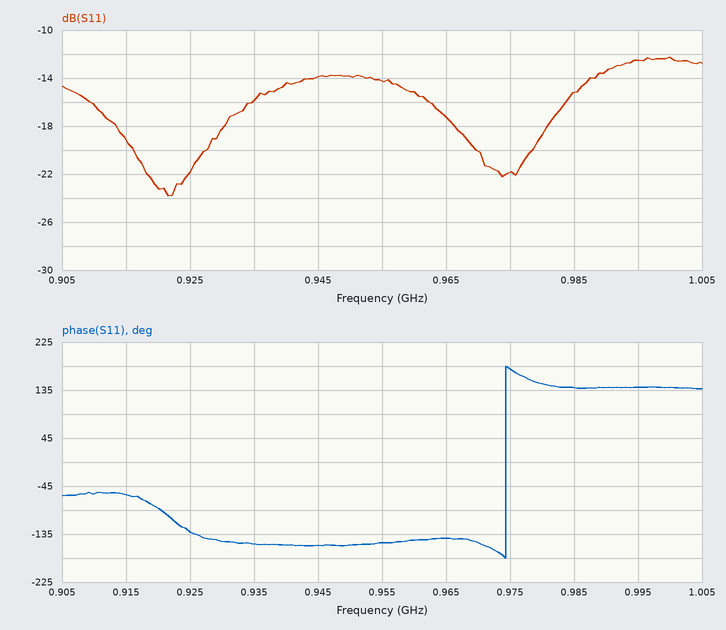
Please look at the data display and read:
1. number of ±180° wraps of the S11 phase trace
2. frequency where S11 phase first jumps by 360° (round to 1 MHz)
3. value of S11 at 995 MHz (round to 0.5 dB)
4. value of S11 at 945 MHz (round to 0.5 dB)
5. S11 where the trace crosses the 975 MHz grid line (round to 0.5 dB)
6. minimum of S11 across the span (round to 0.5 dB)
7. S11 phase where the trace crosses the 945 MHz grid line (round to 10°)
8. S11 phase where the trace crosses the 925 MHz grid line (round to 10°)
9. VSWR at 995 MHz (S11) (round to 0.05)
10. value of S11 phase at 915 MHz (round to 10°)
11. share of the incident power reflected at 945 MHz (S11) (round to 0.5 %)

1
974 MHz
-12.5 dB
-14.0 dB
-22.0 dB
-24.0 dB
-160°
-130°
1.60
-60°
4.0 %
